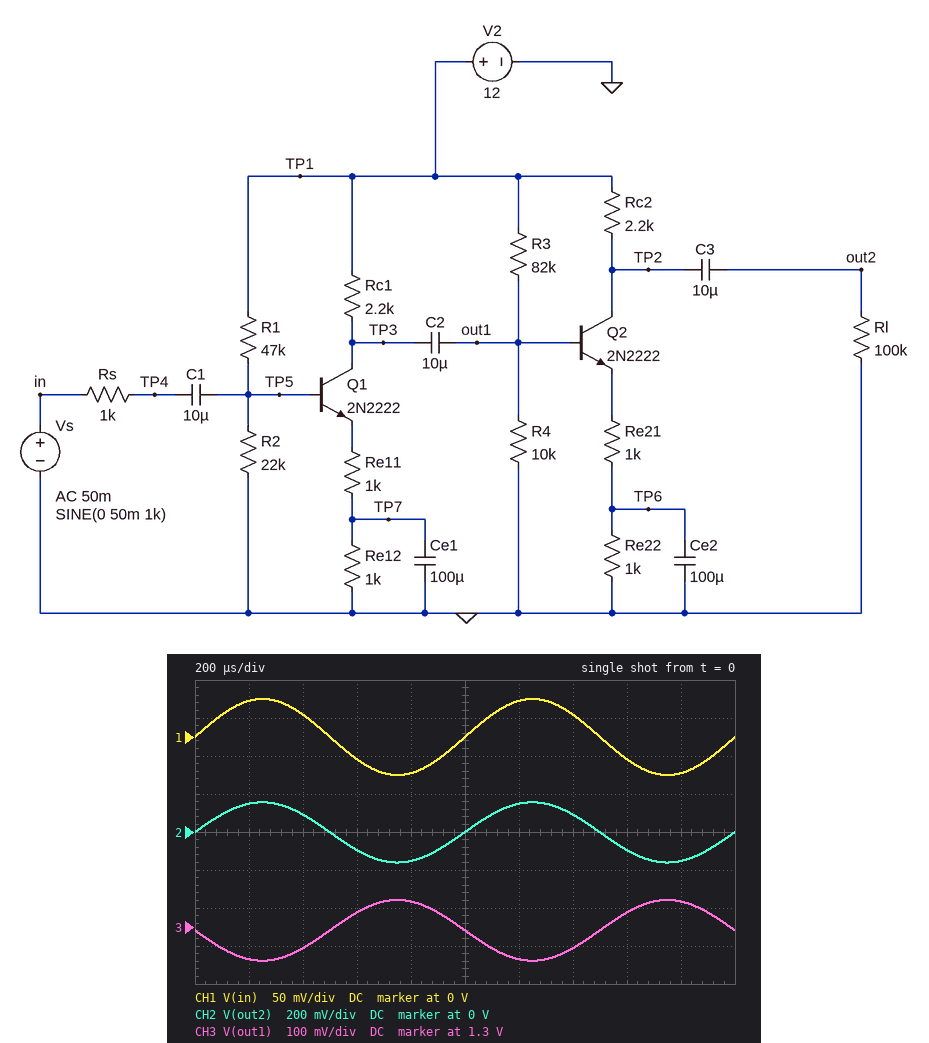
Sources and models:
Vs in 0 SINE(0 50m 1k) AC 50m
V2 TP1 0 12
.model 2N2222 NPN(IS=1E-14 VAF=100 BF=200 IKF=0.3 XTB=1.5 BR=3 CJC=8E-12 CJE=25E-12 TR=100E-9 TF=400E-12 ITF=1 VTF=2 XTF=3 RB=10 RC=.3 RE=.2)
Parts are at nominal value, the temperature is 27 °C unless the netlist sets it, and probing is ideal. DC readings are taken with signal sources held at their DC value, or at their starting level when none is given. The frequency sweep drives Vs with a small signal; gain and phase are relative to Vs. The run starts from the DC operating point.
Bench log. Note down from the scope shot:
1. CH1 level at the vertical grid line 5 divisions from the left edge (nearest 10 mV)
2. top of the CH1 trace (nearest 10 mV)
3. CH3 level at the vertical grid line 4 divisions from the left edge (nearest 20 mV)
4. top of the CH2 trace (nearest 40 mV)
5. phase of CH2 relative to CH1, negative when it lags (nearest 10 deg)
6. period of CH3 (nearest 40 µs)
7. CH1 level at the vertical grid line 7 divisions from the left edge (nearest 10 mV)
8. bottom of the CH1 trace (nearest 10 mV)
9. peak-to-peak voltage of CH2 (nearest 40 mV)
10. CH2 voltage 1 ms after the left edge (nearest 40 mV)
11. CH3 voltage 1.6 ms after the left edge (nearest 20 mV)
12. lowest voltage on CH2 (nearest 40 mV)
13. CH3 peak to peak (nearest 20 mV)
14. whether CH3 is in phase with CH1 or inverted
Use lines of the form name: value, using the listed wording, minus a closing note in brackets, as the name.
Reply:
CH1 level at the vertical grid line 5 divisions from the left edge: 0 V
top of the CH1 trace: 50 mV
CH3 level at the vertical grid line 4 divisions from the left edge: 1.36 V
top of the CH2 trace: 160 mV
phase of CH2 relative to CH1, negative when it lags: 0 deg
period of CH3: 1.00 ms
CH1 level at the vertical grid line 7 divisions from the left edge: 30 mV
bottom of the CH1 trace: -50 mV
peak-to-peak voltage of CH2: 320 mV
CH2 voltage 1 ms after the left edge: 0 V
CH3 voltage 1.6 ms after the left edge: 1.34 V
lowest voltage on CH2: -160 mV
CH3 peak to peak: 160 mV
whether CH3 is in phase with CH1 or inverted: inverted
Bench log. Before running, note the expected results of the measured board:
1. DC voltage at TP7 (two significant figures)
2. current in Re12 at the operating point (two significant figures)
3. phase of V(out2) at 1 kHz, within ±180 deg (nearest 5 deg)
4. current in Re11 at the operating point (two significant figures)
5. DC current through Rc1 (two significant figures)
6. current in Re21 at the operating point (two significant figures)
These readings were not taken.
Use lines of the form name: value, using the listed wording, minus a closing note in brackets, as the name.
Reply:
DC voltage at TP7: 1.5 V
current in Re12 at the operating point: 1.5 mA
phase of V(out2) at 1 kHz, within ±180 deg: 0 deg
current in Re11 at the operating point: 1.5 mA
DC current through Rc1: 1.5 mA
current in Re21 at the operating point: 330 µA
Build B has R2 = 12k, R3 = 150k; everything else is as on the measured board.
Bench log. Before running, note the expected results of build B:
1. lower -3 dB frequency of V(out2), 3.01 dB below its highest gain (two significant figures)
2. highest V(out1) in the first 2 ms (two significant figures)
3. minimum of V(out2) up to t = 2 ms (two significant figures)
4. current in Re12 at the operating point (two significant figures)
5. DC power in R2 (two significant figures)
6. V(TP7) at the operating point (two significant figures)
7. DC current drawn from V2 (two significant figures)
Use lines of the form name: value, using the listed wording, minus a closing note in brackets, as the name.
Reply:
lower -3 dB frequency of V(out2), 3.01 dB below its highest gain: 4.5 Hz
highest V(out1) in the first 2 ms: 820 mV
minimum of V(out2) up to t = 2 ms: -130 mV
current in Re12 at the operating point: 880 µA
DC power in R2: 480 µW
V(TP7) at the operating point: 880 mV
DC current drawn from V2: 1.2 mA
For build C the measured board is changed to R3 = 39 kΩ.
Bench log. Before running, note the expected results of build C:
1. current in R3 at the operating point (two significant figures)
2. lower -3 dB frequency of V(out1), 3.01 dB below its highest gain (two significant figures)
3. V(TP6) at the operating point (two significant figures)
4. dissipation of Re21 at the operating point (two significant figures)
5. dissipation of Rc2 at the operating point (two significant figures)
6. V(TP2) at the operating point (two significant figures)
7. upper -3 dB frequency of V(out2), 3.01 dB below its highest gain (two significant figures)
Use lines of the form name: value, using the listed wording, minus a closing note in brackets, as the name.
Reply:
current in R3 at the operating point: 250 µA
lower -3 dB frequency of V(out1), 3.01 dB below its highest gain: 3.5 Hz
V(TP6) at the operating point: 880 mV
dissipation of Re21 at the operating point: 780 µW
dissipation of Rc2 at the operating point: 1.7 mW
V(TP2) at the operating point: 10 V
upper -3 dB frequency of V(out2), 3.01 dB below its highest gain: 3.8 MHz
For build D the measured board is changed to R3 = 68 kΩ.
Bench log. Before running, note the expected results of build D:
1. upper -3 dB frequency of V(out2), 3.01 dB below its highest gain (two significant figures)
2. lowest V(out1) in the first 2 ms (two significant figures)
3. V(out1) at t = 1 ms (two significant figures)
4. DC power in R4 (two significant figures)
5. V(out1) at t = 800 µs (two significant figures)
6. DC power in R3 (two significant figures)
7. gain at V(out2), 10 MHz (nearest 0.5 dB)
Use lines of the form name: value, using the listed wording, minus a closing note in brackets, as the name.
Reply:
upper -3 dB frequency of V(out2), 3.01 dB below its highest gain: 3.8 MHz
lowest V(out1) in the first 2 ms: 1.4 V
V(out1) at t = 1 ms: 1.5 V
DC power in R4: 230 µW
V(out1) at t = 800 µs: 1.6 V
DC power in R3: 1.6 mW
gain at V(out2), 10 MHz: 1.5 dB
